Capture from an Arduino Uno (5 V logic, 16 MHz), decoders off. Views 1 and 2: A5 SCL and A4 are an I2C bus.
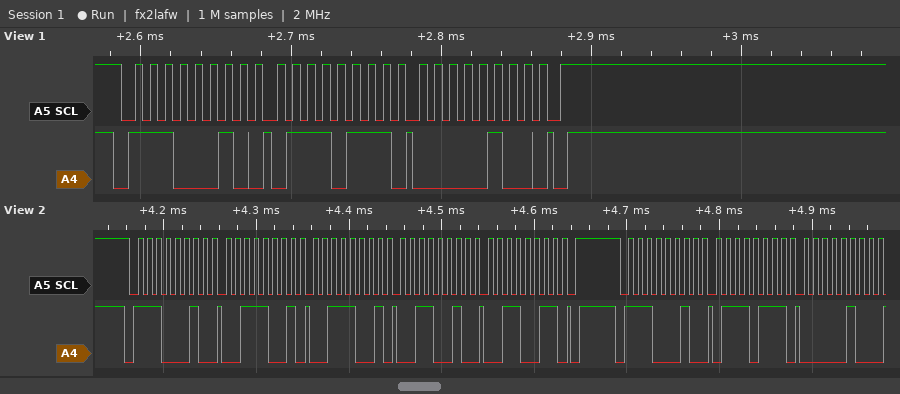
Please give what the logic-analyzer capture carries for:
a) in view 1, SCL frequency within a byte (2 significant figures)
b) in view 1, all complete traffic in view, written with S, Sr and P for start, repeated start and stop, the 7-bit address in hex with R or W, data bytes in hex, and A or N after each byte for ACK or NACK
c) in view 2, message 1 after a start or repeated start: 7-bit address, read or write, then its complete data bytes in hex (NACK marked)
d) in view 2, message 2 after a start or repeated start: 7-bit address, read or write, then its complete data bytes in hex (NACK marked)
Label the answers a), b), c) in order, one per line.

a) 100 kHz
b) S 71W A 77 A 04 A P
c) 0x71 write: 39 39 32 33
d) 0x71 write: 77 04
